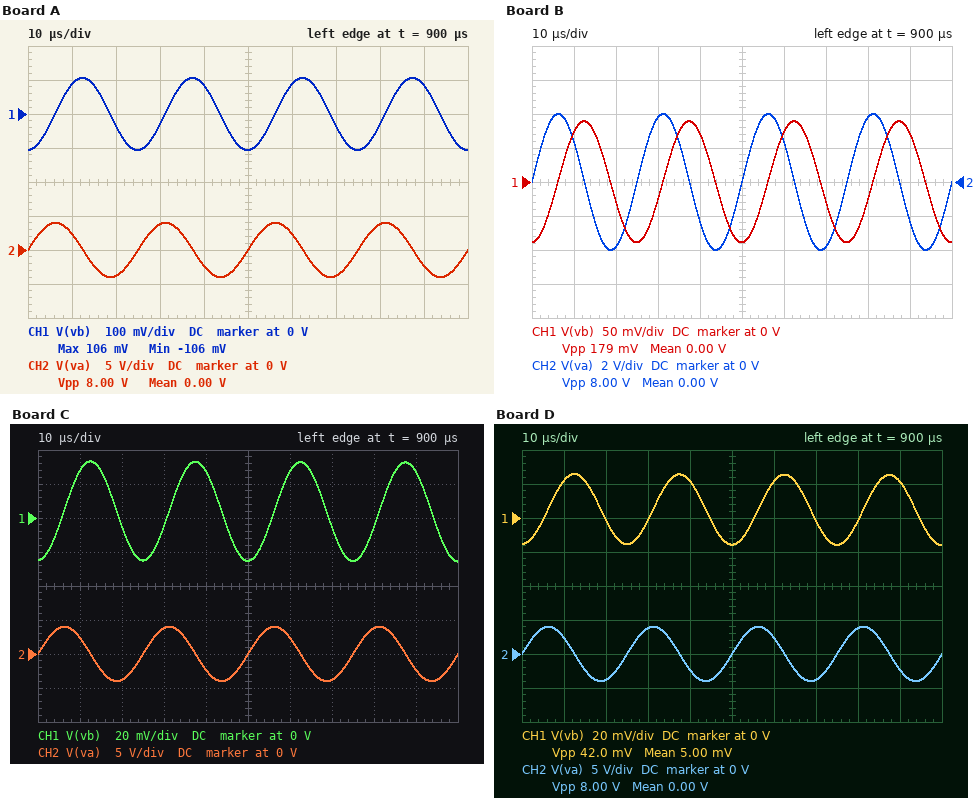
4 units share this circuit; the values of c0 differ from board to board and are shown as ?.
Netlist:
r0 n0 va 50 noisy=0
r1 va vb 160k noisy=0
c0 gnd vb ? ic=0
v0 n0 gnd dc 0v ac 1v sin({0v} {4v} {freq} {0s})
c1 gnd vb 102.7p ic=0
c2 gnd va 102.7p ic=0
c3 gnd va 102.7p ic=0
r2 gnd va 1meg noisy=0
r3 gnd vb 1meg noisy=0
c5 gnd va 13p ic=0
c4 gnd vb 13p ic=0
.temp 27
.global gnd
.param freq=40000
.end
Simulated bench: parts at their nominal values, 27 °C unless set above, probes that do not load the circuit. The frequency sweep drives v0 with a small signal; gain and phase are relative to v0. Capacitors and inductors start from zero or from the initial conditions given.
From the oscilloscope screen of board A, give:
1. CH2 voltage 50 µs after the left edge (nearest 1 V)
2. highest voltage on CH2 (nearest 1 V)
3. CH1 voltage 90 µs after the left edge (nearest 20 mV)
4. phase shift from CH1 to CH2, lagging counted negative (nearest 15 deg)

0 V
4 V
80 mV
90 deg
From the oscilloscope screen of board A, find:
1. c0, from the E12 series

820 pF
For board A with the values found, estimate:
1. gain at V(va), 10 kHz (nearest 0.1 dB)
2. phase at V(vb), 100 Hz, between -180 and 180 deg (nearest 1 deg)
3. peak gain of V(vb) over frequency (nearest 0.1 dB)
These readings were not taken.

0 dB
-5 deg
-1.3 dB
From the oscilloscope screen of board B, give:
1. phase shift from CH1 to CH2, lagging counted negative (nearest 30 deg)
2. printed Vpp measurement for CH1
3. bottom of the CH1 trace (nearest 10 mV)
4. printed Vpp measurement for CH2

90 deg
179 mV
-90 mV
8.00 V
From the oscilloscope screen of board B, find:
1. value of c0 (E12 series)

1 nF
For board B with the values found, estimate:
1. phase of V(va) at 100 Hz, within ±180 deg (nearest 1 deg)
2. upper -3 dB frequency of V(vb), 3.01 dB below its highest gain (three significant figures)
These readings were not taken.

0 deg
1.03 kHz
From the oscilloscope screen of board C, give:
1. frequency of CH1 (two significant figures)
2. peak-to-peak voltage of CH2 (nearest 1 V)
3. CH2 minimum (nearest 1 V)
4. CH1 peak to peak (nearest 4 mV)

40 kHz
8 V
-4 V
60 mV
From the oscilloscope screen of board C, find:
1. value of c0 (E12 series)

3.3 nF
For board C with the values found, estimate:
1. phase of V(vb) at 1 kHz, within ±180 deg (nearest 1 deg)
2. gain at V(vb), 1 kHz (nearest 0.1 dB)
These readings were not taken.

-71 deg
-11.2 dB
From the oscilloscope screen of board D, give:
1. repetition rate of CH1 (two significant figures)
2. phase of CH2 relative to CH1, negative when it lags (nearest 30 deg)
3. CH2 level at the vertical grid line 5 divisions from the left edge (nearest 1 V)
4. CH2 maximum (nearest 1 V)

40 kHz
90 deg
0 V
4 V
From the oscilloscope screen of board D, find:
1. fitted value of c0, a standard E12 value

4.7 nF
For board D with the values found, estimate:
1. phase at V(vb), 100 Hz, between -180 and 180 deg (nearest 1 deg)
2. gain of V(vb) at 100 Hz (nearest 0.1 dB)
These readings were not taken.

-23 deg
-2.0 dB
